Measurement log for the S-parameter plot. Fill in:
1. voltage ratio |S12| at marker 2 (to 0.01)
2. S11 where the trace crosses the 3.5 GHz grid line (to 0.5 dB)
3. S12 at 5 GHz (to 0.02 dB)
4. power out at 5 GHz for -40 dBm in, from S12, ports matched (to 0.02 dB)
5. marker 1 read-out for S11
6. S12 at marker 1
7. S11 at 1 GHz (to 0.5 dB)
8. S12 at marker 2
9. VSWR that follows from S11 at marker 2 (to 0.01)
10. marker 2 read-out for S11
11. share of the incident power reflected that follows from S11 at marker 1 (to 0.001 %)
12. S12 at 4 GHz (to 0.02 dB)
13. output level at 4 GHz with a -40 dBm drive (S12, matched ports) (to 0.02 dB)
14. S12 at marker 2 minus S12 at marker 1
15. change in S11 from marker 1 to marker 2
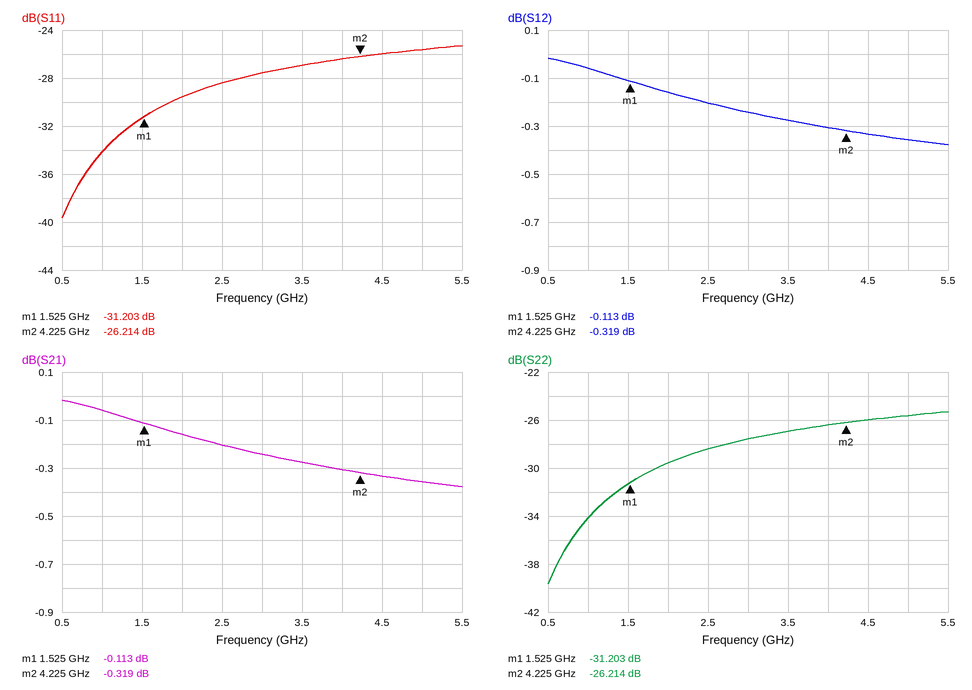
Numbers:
0.96
-27.0 dB
-0.36 dB
-40.36 dBm
-31.203 dB
-0.113 dB
-34.0 dB
-0.319 dB
1.10
-26.214 dB
0.076 %
-0.30 dB
-40.30 dBm
-0.206 dB
4.989 dB
